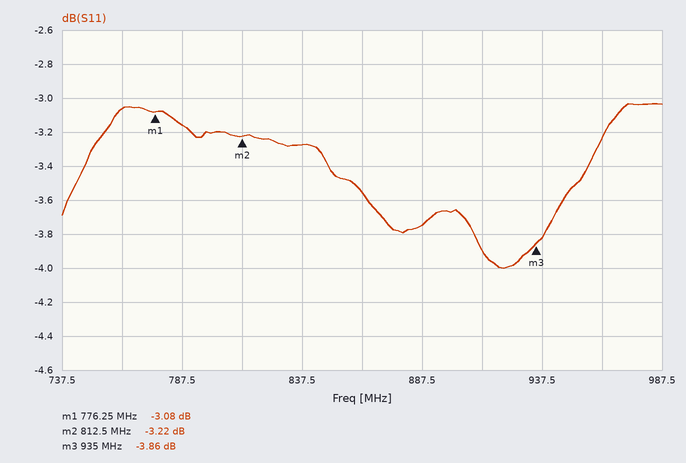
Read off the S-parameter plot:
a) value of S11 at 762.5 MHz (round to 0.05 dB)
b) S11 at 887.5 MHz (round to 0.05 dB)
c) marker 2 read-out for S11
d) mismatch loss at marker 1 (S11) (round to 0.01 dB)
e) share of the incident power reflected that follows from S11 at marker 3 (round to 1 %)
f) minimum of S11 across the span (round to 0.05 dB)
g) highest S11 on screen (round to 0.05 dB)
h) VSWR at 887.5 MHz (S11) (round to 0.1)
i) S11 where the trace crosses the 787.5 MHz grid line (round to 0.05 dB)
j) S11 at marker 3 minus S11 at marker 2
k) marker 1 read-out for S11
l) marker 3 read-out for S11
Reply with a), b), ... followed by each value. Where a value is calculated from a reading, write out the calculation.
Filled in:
a) -3.05 dB
b) -3.75 dB
c) -3.22 dB
d) −10 log10(1 − 10^(-3.08/10)) ≈ 2.94 dB
e) 10^(-3.86/10) ≈ 41 %
f) -4.00 dB
g) -3.05 dB
h) |Γ| = 10^(-3.75/20) = 0.6494; VSWR = (1 + 0.6494)/(1 − 0.6494) ≈ 4.7
i) -3.15 dB
j) -3.86 − (-3.22) = -0.64 dB
k) -3.08 dB
l) -3.86 dB
